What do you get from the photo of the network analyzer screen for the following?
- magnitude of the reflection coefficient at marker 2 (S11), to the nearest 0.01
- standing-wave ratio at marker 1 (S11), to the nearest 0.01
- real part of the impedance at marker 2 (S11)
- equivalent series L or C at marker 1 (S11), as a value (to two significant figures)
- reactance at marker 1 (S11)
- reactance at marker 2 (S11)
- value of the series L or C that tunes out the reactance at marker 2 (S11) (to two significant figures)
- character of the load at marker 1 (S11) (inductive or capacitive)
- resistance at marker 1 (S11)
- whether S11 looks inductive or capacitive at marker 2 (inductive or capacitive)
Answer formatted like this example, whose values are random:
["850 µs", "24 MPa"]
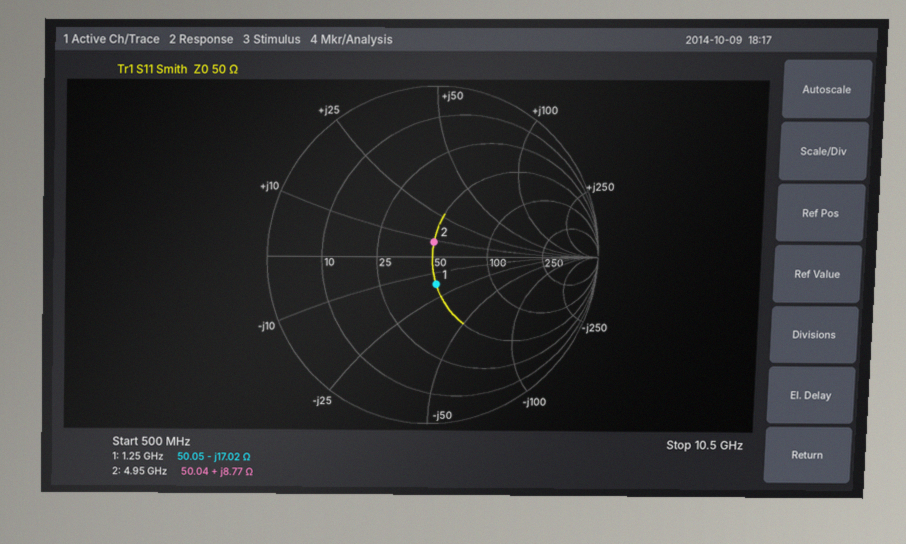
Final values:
["0.09", "1.40", "50.04 Ω", "7.5 pF", "-17.02 Ω", "+8.77 Ω", "3.7 pF", "capacitive", "50.05 Ω", "inductive"]
